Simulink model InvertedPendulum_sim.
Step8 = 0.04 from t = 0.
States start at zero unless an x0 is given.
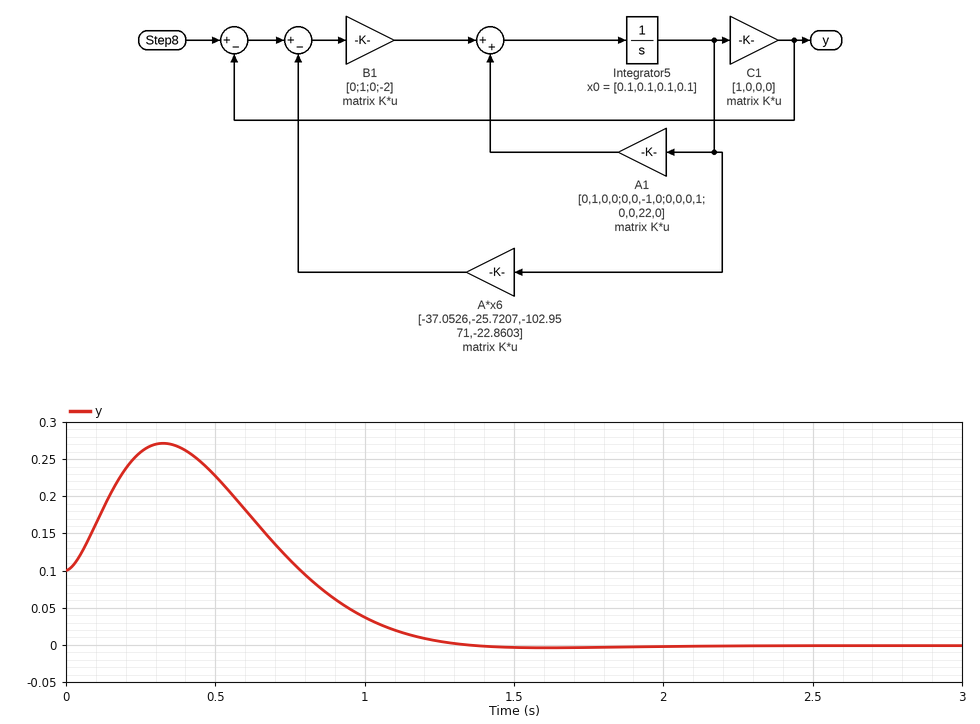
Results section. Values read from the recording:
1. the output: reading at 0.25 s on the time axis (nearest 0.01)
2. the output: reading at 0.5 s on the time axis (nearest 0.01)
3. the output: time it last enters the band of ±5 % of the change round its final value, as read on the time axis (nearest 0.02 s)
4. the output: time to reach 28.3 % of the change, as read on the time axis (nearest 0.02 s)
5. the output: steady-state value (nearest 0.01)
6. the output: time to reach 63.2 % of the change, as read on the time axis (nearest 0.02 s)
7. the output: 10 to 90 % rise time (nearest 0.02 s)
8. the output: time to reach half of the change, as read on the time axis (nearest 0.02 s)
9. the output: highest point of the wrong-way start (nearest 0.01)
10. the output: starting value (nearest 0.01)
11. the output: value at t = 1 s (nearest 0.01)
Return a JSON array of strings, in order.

["0.26", "0.23", "1.26 s", "0.86 s", "0.00", "1.00 s", "0.38 s", "0.94 s", "0.27", "0.10", "0.04"]
